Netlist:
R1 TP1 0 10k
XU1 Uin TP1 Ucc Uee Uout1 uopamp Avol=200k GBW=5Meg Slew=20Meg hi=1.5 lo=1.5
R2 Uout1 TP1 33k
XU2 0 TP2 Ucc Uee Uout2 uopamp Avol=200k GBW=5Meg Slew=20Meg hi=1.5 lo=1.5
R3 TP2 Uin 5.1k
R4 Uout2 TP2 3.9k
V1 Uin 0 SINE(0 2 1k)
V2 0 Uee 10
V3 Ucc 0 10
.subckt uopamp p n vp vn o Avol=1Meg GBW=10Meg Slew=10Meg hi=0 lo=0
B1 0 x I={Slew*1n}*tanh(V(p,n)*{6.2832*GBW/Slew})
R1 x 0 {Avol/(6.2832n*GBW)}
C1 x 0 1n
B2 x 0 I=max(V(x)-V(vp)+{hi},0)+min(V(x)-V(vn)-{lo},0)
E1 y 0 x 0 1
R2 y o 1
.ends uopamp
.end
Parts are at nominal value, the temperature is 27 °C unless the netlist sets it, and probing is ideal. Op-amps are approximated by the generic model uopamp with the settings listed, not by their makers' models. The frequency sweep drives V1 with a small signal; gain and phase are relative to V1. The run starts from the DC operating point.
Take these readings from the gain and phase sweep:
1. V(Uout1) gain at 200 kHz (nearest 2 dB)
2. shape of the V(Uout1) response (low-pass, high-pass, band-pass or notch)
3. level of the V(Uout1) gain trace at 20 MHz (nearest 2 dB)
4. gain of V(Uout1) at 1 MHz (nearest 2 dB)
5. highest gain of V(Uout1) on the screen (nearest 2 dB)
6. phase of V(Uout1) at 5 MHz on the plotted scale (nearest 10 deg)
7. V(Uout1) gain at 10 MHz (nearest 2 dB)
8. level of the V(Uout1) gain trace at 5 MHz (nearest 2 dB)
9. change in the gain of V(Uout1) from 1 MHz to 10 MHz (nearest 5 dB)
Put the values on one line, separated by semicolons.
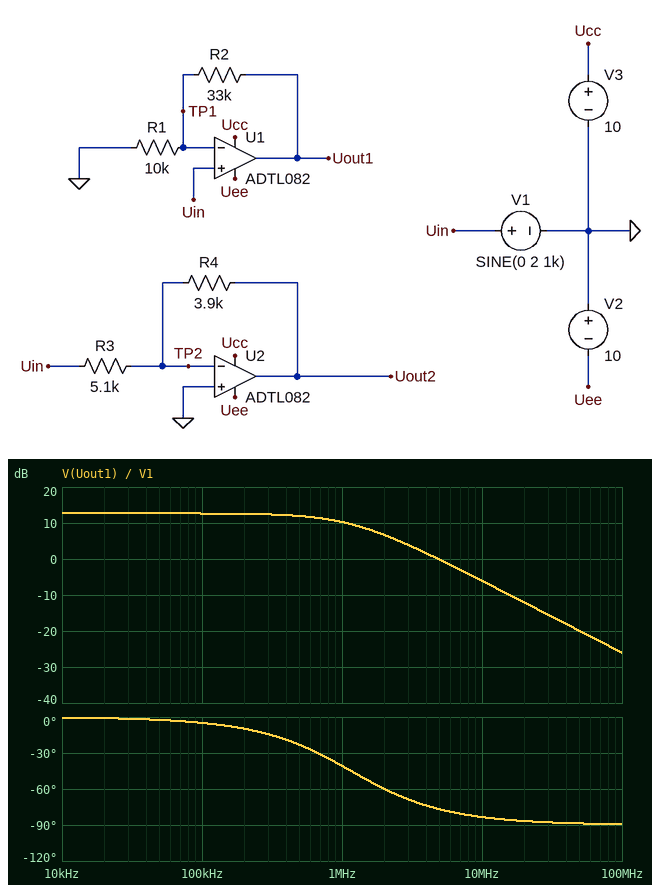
12 dB; low-pass; -12 dB; 10 dB; 12 dB; -80 deg; -6 dB; 0 dB; -15 dB
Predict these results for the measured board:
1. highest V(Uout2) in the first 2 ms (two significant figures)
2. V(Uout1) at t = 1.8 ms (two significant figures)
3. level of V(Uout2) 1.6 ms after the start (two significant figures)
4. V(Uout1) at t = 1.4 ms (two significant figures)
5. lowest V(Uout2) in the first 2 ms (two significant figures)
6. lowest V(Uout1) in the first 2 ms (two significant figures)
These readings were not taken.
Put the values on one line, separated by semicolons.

1.5 V; -8.2 V; 900 mV; 5.1 V; -1.5 V; -8.5 V
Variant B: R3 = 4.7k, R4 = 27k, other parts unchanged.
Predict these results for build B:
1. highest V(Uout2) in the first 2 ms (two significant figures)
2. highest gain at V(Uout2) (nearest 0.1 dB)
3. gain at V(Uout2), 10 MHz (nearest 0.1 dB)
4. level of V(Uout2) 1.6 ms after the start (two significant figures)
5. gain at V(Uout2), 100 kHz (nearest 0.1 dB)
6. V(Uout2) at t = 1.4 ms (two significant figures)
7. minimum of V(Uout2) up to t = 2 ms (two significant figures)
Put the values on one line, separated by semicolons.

8.5 V; 15.2 dB; -7.4 dB; 6.7 V; 15.1 dB; -6.8 V; -8.5 V
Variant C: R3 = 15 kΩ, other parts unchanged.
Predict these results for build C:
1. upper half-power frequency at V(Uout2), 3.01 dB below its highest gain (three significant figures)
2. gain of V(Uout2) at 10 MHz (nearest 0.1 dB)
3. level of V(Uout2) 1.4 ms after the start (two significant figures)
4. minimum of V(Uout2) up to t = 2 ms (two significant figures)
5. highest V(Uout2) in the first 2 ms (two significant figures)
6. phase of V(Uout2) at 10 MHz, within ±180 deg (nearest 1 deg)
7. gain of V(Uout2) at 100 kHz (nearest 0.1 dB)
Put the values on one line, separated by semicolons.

3.97 MHz; -20.4 dB; -310 mV; -520 mV; 520 mV; 112 deg; -11.7 dB
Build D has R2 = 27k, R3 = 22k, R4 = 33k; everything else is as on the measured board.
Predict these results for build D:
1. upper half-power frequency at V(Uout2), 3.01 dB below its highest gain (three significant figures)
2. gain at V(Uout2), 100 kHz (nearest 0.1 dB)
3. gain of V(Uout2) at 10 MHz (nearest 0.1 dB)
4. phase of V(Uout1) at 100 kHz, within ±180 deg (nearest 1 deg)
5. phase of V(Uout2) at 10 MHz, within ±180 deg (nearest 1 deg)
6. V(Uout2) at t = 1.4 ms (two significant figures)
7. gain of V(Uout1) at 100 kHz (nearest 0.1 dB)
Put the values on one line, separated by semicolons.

2.00 MHz; 3.5 dB; -10.6 dB; -4 deg; 101 deg; -1.8 V; 11.3 dB
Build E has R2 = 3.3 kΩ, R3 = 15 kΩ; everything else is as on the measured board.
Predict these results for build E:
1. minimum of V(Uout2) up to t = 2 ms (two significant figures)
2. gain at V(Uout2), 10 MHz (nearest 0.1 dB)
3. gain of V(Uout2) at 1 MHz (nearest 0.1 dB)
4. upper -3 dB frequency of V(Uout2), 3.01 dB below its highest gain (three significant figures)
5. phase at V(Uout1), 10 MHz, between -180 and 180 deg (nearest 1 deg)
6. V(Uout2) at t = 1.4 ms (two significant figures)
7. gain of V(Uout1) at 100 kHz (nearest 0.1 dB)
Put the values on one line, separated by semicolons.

-520 mV; -20.4 dB; -12.0 dB; 3.97 MHz; -69 deg; -310 mV; 2.5 dB
